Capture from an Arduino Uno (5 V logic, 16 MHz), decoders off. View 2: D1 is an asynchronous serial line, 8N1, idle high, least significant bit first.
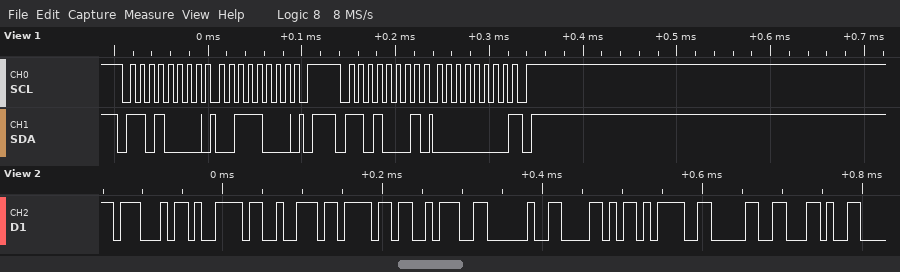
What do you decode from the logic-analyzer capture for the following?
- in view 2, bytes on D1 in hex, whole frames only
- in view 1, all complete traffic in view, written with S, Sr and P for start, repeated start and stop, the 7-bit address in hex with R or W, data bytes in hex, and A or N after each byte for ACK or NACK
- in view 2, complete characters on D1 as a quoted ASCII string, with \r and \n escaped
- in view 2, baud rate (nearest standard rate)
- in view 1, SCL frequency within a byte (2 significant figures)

47 79 72 6F 3A 20 58 3D 30 2C
S 68W A 38 A P S 68R A 00 N P
"Gyro: X=0,"
115200 baud
100 kHz
